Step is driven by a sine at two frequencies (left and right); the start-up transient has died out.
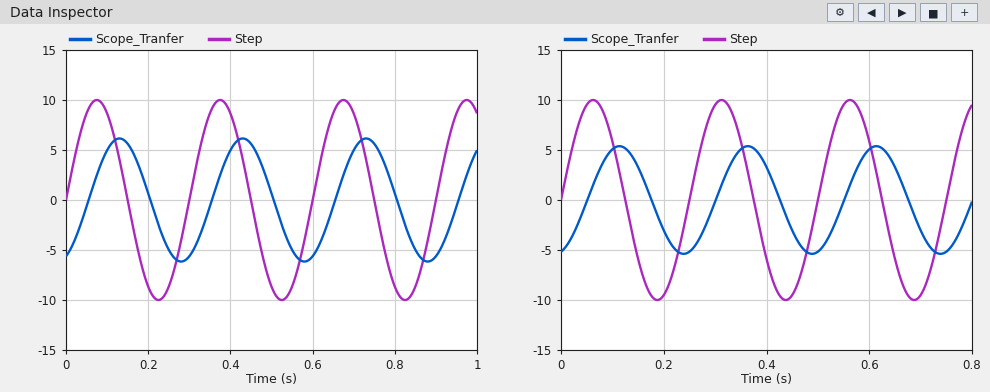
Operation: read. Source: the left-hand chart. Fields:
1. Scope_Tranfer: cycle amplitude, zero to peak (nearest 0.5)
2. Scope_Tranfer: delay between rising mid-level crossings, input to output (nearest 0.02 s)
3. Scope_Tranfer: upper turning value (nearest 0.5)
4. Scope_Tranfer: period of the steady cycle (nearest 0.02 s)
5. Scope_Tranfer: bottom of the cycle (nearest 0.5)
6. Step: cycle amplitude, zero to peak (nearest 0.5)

6.0
0.06 s
6.0
0.30 s
-6.0
10.0
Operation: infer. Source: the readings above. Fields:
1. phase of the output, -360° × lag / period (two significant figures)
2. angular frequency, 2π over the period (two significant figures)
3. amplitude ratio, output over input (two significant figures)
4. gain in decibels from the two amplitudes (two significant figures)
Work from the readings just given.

-72°
21 rad/s
0.60
-4.4 dB
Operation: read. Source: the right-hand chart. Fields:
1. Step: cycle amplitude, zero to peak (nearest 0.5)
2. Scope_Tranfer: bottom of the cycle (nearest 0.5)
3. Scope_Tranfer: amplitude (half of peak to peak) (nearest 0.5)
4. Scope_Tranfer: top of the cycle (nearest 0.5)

10.0
-5.5
5.5
5.5
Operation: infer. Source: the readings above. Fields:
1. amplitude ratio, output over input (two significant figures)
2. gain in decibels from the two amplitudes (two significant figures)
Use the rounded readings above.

0.55
-5.2 dB
